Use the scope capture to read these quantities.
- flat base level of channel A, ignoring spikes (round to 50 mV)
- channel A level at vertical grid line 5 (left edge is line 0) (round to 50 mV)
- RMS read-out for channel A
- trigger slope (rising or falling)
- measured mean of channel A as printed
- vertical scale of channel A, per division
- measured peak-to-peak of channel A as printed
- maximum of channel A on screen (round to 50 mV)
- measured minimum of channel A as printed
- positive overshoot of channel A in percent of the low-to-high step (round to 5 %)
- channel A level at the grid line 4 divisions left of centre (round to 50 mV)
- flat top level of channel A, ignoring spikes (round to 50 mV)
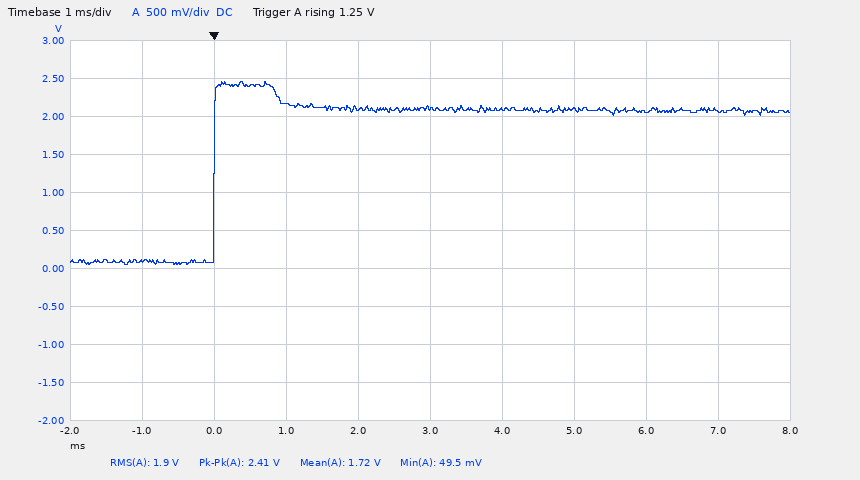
100 mV
2.10 V
1.9 V
rising
1.72 V
500 mV
2.41 V
2.45 V
49.5 mV
20 %
100 mV
2.10 V
